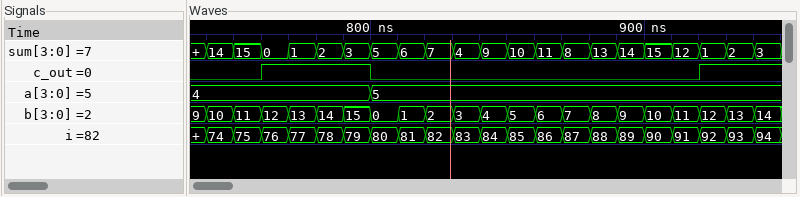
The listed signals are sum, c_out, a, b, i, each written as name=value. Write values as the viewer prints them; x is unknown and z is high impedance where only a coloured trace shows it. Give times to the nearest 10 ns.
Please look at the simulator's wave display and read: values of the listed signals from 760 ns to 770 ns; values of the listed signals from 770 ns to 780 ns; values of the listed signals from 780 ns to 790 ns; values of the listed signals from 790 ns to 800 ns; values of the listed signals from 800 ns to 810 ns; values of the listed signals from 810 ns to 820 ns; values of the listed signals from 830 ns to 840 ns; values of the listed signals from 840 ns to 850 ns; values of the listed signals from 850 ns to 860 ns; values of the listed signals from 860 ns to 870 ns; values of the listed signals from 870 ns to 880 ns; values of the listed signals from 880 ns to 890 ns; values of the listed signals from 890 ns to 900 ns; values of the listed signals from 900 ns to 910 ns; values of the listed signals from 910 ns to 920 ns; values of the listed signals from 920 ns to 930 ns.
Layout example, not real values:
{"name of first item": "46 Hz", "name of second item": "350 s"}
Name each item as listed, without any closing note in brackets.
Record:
{"values of the listed signals from 760 ns to 770 ns": "sum=0, c_out=1, a=4, b=12, i=76", "values of the listed signals from 770 ns to 780 ns": "sum=1, c_out=1, a=4, b=13, i=77", "values of the listed signals from 780 ns to 790 ns": "sum=2, c_out=1, a=4, b=14, i=78", "values of the listed signals from 790 ns to 800 ns": "sum=3, c_out=1, a=4, b=15, i=79", "values of the listed signals from 800 ns to 810 ns": "sum=5, c_out=0, a=5, b=0, i=80", "values of the listed signals from 810 ns to 820 ns": "sum=6, c_out=0, a=5, b=1, i=81", "values of the listed signals from 830 ns to 840 ns": "sum=4, c_out=0, a=5, b=3, i=83", "values of the listed signals from 840 ns to 850 ns": "sum=9, c_out=0, a=5, b=4, i=84", "values of the listed signals from 850 ns to 860 ns": "sum=10, c_out=0, a=5, b=5, i=85", "values of the listed signals from 860 ns to 870 ns": "sum=11, c_out=0, a=5, b=6, i=86", "values of the listed signals from 870 ns to 880 ns": "sum=8, c_out=0, a=5, b=7, i=87", "values of the listed signals from 880 ns to 890 ns": "sum=13, c_out=0, a=5, b=8, i=88", "values of the listed signals from 890 ns to 900 ns": "sum=14, c_out=0, a=5, b=9, i=89", "values of the listed signals from 900 ns to 910 ns": "sum=15, c_out=0, a=5, b=10, i=90", "values of the listed signals from 910 ns to 920 ns": "sum=12, c_out=0, a=5, b=11, i=91", "values of the listed signals from 920 ns to 930 ns": "sum=1, c_out=1, a=5, b=12, i=92"}
